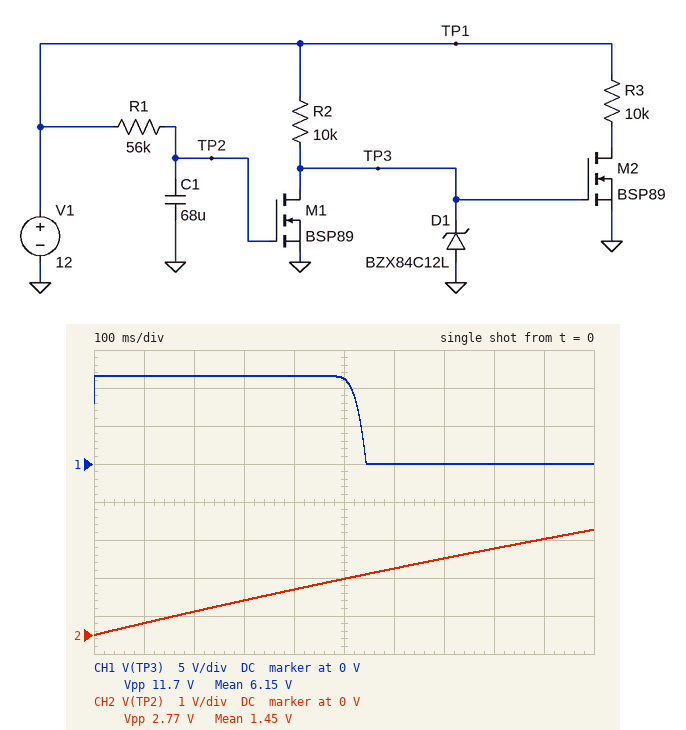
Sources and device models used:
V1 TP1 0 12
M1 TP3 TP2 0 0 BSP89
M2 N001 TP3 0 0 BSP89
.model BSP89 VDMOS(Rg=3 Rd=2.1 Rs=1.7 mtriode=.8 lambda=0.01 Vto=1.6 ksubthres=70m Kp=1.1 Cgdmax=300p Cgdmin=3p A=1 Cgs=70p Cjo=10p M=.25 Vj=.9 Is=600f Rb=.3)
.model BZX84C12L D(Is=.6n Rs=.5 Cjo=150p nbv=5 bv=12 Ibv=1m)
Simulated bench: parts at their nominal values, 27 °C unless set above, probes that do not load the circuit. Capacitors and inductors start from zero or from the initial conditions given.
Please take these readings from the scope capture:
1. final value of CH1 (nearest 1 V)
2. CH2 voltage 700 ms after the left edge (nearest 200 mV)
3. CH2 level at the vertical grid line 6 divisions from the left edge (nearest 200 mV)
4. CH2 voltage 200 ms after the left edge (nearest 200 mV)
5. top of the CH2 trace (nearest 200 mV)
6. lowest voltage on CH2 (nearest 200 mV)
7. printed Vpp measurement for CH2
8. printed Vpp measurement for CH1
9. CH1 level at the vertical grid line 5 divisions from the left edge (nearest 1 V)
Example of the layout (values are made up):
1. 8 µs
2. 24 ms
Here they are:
1. 0 V
2. 2.0 V
3. 1.8 V
4. 600 mV
5. 2.8 V
6. 0 V
7. 2.77 V
8. 11.7 V
9. 11 V
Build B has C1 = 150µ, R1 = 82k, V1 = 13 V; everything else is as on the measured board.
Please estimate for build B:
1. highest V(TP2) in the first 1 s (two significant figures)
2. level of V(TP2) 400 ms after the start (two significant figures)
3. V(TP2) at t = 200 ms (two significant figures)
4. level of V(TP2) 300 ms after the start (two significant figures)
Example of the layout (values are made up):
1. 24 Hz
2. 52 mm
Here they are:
1. 1.0 V
2. 420 mV
3. 210 mV
4. 310 mV
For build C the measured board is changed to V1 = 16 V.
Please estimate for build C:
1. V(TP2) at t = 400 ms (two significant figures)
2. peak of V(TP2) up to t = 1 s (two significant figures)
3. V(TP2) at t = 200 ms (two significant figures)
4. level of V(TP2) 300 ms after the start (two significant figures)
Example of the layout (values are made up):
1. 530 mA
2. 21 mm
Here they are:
1. 1.6 V
2. 3.7 V
3. 820 mV
4. 1.2 V
